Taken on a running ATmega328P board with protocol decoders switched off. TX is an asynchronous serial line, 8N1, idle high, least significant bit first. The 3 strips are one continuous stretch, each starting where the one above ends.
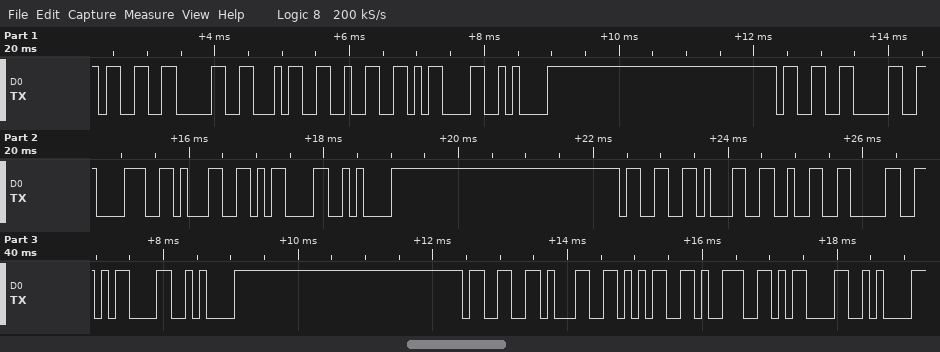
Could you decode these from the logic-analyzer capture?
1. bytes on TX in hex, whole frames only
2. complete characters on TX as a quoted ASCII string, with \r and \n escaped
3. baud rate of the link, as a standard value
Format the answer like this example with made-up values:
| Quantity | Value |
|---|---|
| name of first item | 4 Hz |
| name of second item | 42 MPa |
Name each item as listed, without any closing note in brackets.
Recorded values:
| Quantity | Value |
|---|---|
| bytes on TX in hex, whole frames only | 33 30 34 32 0D 0A 33 30 38 31 0D 0A 33 31 32 30 0D 0A 33 31 35 39 0D 0A |
| complete characters on TX as a quoted ASCII string, with \r and \n escaped | "3042\r\n3081\r\n3120\r\n3159\r\n" |
| baud rate of the link, as a standard value | 9600 baud |
